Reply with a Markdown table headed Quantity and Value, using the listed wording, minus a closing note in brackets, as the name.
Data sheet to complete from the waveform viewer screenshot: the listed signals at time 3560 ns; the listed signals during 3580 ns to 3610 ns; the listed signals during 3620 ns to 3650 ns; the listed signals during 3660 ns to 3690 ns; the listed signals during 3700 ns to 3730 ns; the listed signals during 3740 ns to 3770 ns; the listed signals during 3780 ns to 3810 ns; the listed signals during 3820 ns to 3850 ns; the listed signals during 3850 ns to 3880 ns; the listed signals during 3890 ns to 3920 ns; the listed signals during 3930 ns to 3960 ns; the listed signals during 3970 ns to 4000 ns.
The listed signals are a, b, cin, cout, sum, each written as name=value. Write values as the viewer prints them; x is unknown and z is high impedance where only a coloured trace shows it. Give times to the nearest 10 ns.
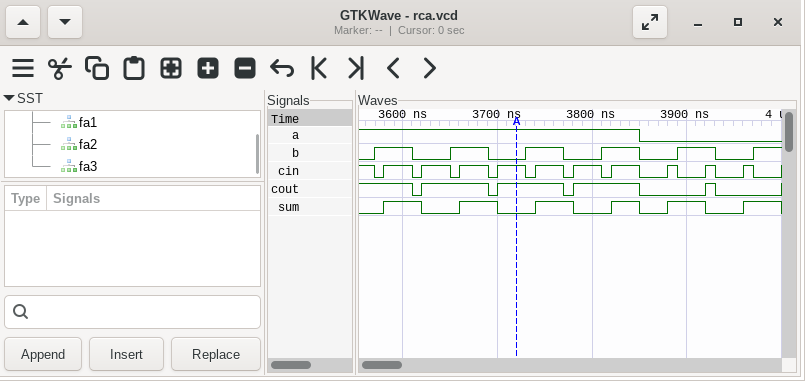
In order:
| Quantity | Value |
|---|---|
| the listed signals at time 3560 ns | a=1, b=0, cin=1, cout=1, sum=0 |
| the listed signals during 3580 ns to 3610 ns | a=1, b=1, cin=1, cout=1, sum=1 |
| the listed signals during 3620 ns to 3650 ns | a=1, b=0, cin=1, cout=1, sum=0 |
| the listed signals during 3660 ns to 3690 ns | a=1, b=1, cin=1, cout=1, sum=1 |
| the listed signals during 3700 ns to 3730 ns | a=1, b=0, cin=1, cout=1, sum=0 |
| the listed signals during 3740 ns to 3770 ns | a=1, b=1, cin=1, cout=1, sum=1 |
| the listed signals during 3780 ns to 3810 ns | a=1, b=0, cin=1, cout=1, sum=0 |
| the listed signals during 3820 ns to 3850 ns | a=1, b=1, cin=1, cout=1, sum=1 |
| the listed signals during 3850 ns to 3880 ns | a=0, b=0, cin=0, cout=0, sum=0 |
| the listed signals during 3890 ns to 3920 ns | a=0, b=1, cin=0, cout=0, sum=1 |
| the listed signals during 3930 ns to 3960 ns | a=0, b=0, cin=0, cout=0, sum=0 |
| the listed signals during 3970 ns to 4000 ns | a=0, b=1, cin=0, cout=0, sum=1 |
